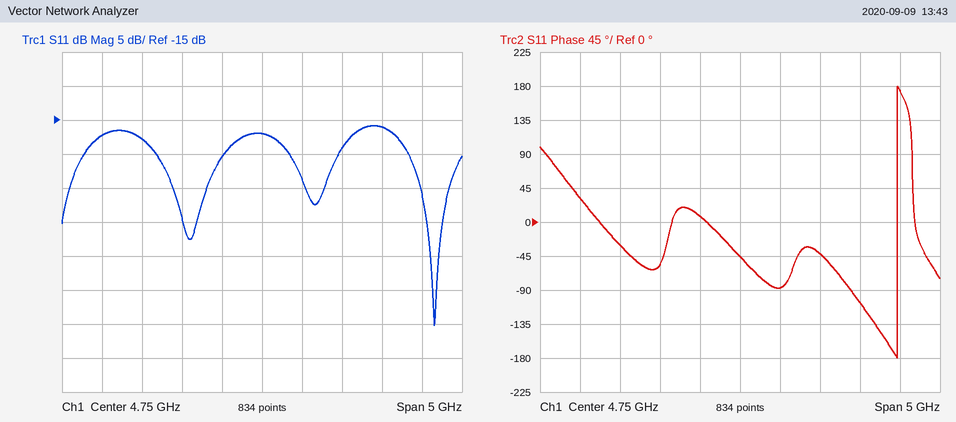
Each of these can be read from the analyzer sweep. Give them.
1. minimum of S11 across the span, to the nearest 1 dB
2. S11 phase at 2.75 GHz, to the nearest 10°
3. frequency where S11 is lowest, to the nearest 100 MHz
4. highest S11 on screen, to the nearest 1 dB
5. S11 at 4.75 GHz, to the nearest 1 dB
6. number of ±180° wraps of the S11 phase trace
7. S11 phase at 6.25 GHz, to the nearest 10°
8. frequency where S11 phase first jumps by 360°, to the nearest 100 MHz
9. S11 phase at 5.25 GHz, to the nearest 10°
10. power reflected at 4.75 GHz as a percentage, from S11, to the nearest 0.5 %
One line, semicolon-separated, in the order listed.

-45 dB; 30°; 6.9 GHz; -16 dB; -17 dB; 1; -110°; 6.7 GHz; -90°; 2.0 %
